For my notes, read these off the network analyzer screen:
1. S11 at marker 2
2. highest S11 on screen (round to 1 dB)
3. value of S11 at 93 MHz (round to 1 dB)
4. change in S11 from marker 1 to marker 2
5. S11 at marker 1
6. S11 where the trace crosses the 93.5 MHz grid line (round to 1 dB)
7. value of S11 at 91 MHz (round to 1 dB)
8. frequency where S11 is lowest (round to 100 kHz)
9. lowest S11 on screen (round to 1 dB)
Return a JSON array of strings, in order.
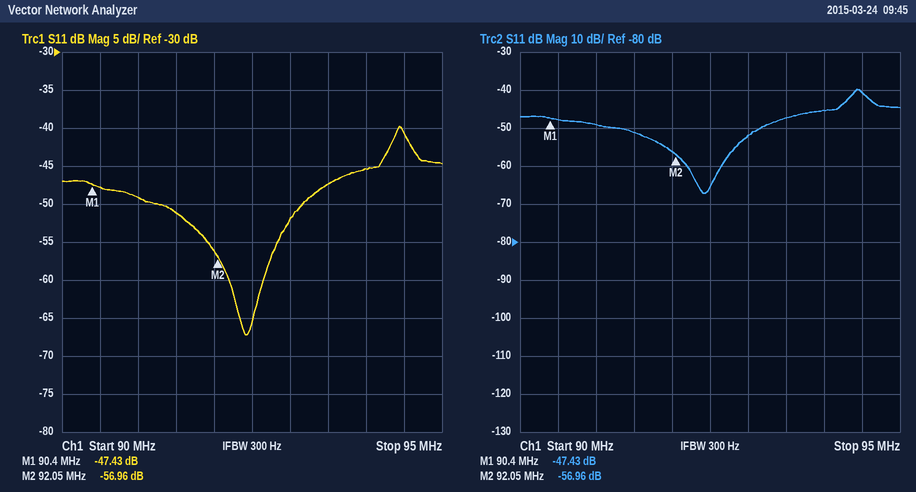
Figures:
["-56.96 dB", "-40 dB", "-52 dB", "-9.53 dB", "-47.43 dB", "-47 dB", "-49 dB", "92.4 MHz", "-67 dB"]
